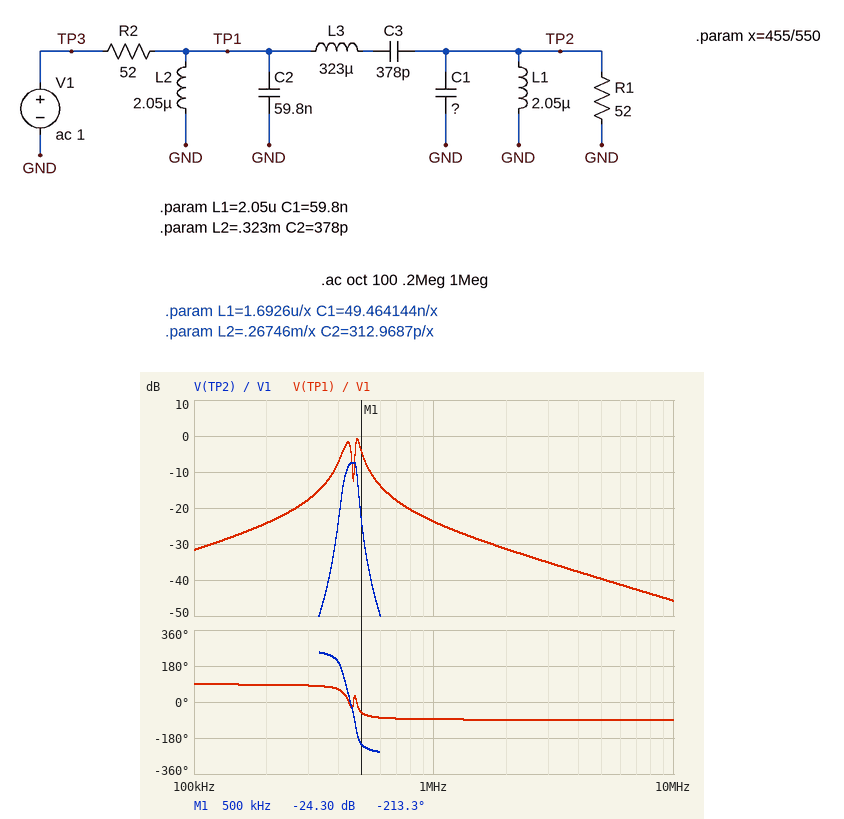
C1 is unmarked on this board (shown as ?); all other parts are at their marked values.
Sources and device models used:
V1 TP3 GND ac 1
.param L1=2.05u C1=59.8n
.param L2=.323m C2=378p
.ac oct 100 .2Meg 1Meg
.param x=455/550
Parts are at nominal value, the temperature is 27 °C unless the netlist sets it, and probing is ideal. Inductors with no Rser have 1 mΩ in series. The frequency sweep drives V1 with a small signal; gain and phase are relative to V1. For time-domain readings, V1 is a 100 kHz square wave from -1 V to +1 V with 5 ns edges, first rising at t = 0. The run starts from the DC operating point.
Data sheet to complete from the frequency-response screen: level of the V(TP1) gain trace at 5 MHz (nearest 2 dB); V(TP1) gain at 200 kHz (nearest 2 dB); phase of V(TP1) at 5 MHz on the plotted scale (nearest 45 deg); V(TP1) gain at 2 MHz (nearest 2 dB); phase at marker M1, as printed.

-40 dB
-24 dB
-90 deg
-32 dB
-213.3 deg
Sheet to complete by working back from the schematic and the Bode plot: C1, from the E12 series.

68 nF
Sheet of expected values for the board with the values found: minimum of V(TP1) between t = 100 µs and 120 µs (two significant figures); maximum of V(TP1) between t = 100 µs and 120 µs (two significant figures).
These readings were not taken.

-220 mV
220 mV
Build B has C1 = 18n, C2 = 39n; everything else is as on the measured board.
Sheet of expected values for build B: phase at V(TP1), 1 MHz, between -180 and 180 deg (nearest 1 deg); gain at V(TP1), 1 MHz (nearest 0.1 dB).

-83 deg
-18.8 dB
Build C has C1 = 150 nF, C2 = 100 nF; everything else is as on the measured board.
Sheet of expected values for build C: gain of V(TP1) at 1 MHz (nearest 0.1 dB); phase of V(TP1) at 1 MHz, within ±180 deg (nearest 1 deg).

-29.1 dB
-88 deg
